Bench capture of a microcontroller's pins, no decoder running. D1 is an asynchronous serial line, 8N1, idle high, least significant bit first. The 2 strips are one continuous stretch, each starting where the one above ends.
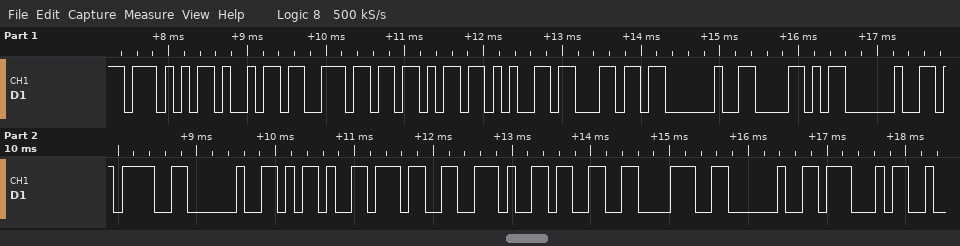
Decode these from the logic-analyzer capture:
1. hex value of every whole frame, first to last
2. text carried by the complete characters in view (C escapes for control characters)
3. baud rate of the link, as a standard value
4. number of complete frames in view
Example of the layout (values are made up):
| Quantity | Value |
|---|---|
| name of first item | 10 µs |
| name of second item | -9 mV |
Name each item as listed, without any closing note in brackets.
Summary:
| Quantity | Value |
|---|---|
| hex value of every whole frame, first to last | 57 69 6E 6B 65 6C 20 58 20 3D 20 2D 37 2E 33 38 20 47 |
| text carried by the complete characters in view | "Winkel X = -7.38 G" |
| baud rate of the link, as a standard value | 9600 baud |
| number of complete frames in view | 18 |
